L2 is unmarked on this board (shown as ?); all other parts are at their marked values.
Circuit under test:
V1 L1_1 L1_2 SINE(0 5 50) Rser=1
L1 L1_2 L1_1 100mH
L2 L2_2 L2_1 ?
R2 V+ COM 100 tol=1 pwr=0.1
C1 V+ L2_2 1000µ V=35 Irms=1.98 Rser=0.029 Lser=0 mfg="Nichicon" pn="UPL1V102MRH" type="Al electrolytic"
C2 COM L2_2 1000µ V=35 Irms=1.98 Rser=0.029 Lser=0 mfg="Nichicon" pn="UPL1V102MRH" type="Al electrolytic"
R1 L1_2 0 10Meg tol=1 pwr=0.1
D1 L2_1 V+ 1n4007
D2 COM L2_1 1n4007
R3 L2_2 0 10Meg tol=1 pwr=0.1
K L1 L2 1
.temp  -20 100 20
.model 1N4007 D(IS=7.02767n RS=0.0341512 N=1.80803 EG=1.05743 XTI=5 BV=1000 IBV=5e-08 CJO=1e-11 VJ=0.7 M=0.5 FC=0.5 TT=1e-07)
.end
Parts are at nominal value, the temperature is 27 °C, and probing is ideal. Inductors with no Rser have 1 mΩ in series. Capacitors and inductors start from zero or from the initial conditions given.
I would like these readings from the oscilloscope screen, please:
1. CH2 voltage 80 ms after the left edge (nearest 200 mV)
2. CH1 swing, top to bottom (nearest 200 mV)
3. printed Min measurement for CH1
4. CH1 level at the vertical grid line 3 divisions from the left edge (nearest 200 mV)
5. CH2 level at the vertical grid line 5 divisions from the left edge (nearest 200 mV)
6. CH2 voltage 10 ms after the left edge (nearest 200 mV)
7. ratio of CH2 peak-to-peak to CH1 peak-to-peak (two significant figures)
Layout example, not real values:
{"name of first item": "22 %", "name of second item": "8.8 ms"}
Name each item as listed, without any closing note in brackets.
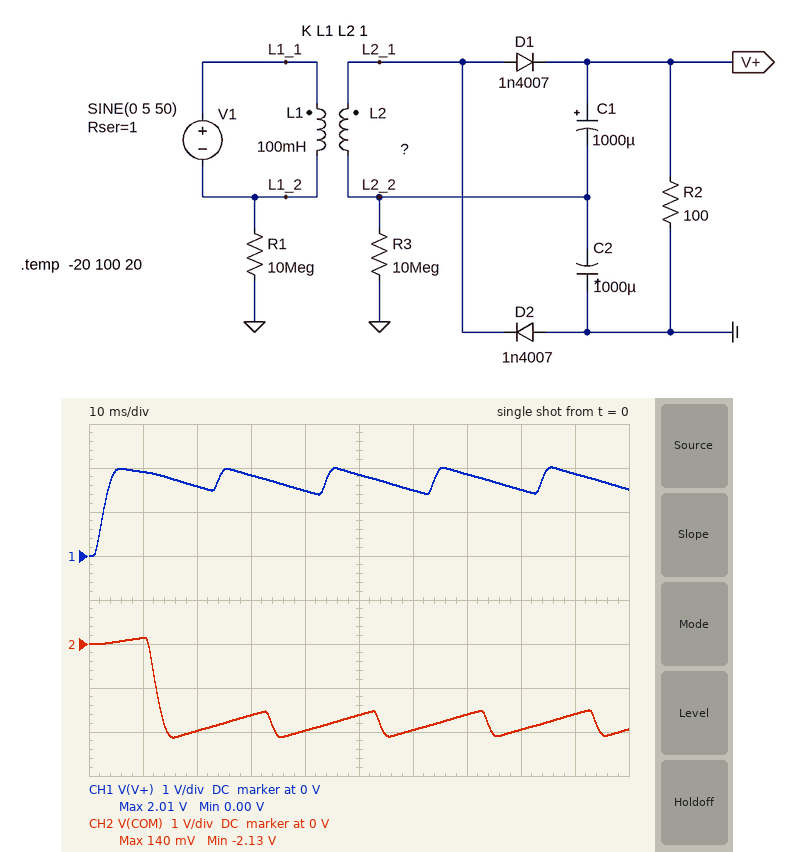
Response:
{"CH2 voltage 80 ms after the left edge": "-2.0 V", "CH1 swing, top to bottom": "2.0 V", "printed Min measurement for CH1": "0.00 V", "CH1 level at the vertical grid line 3 divisions from the left edge": "1.8 V", "CH2 level at the vertical grid line 5 divisions from the left edge": "-1.6 V", "CH2 voltage 10 ms after the left edge": "200 mV", "ratio of CH2 peak-to-peak to CH1 peak-to-peak": "1.1"}
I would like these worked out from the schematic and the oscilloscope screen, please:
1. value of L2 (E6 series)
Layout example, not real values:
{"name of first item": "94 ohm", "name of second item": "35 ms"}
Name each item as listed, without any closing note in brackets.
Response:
{"value of L2": "33 mH"}
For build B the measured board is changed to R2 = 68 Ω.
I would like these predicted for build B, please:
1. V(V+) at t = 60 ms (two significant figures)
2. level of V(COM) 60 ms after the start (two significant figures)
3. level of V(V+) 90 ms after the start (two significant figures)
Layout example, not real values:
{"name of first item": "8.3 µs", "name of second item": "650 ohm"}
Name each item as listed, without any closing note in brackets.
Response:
{"V(V+) at t = 60 ms": "1.3 V", "level of V(COM) 60 ms after the start": "-1.9 V", "level of V(V+) 90 ms after the start": "1.8 V"}
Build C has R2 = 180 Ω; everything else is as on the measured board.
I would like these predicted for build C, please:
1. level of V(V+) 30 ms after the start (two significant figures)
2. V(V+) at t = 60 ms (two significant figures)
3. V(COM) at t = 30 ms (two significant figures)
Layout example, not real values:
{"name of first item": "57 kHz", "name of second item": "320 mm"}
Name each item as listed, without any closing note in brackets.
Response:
{"level of V(V+) 30 ms after the start": "1.9 V", "V(V+) at t = 60 ms": "1.7 V", "V(COM) at t = 30 ms": "-1.8 V"}
